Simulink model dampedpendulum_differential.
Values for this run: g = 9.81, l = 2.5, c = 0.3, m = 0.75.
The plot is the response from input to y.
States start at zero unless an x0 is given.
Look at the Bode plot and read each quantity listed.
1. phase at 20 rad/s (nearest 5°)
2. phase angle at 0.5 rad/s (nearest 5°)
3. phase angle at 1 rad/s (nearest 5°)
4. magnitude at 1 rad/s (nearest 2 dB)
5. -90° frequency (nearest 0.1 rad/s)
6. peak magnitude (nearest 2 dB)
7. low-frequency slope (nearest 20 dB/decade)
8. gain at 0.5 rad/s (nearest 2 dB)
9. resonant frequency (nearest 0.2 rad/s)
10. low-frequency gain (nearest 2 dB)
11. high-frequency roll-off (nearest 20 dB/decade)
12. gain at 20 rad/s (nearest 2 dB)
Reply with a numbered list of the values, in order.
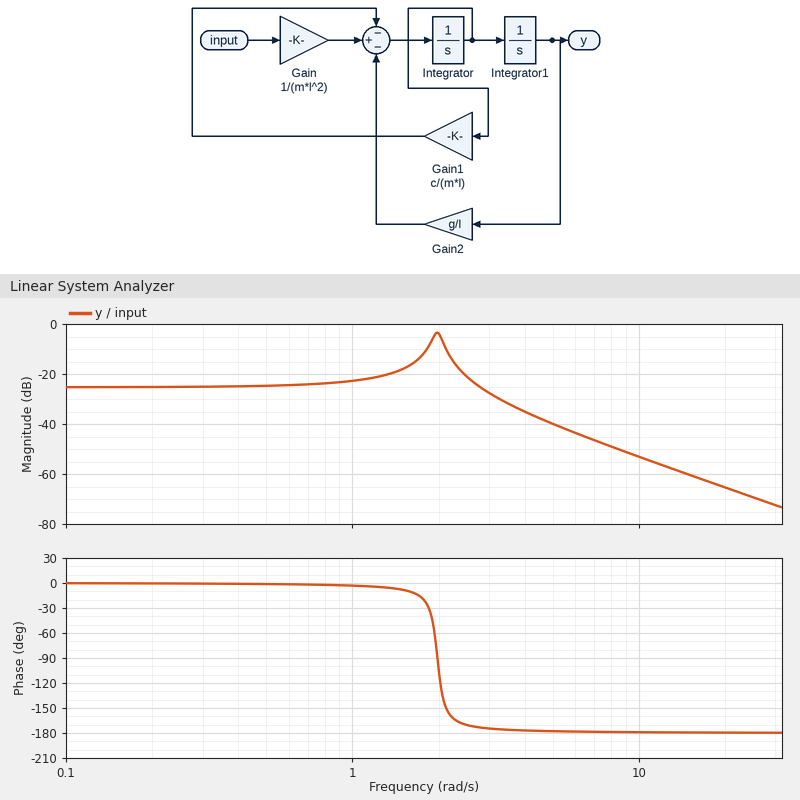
1. -180°
2. 0°
3. -5°
4. -22 dB
5. 2.0 rad/s
6. -4 dB
7. 0 dB/decade
8. -24 dB
9. 2.0 rad/s
10. -26 dB
11. -40 dB/decade
12. -66 dB
